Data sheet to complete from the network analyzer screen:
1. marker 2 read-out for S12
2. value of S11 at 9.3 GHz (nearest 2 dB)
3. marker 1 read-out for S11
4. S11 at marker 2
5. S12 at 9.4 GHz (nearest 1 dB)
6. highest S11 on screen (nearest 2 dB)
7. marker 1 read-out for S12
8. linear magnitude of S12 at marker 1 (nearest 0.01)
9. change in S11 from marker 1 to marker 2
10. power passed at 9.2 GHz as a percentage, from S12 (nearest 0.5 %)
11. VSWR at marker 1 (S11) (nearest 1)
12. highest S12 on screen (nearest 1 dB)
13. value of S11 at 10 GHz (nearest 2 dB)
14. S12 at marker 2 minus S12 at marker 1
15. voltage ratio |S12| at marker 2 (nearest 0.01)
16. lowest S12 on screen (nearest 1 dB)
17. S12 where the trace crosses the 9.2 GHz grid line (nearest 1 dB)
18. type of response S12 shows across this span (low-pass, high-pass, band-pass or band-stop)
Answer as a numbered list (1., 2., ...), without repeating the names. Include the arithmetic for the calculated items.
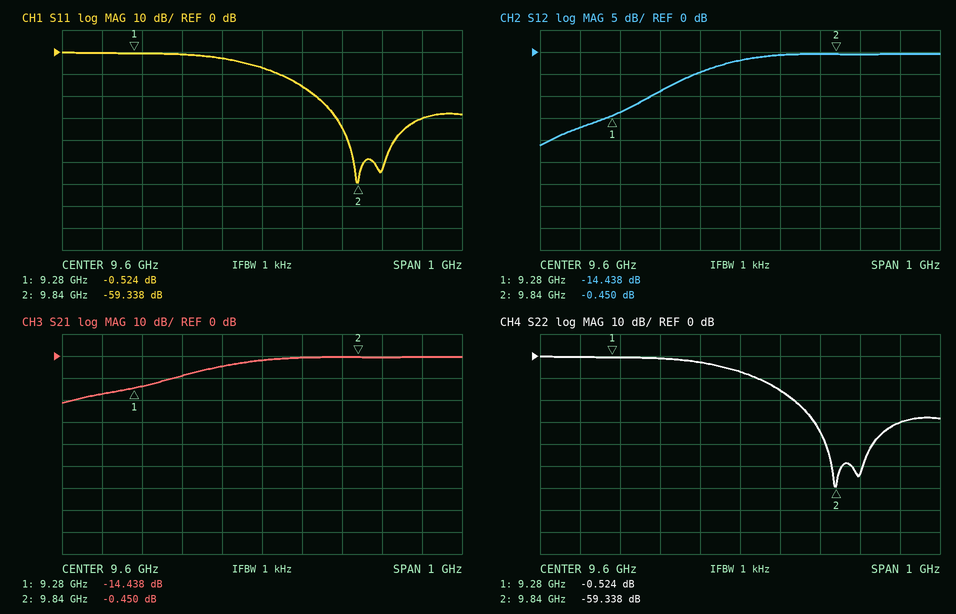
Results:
1. -0.450 dB
2. 0 dB
3. -0.524 dB
4. -59.338 dB
5. -9 dB
6. 0 dB
7. -14.438 dB
8. 10^(-14.438/20) ≈ 0.19
9. -59.338 − (-0.524) = -58.814 dB
10. 10^(-17/10) ≈ 2.0 %
11. (1 + 0.9415)/(1 − 0.9415) ≈ 33
12. 0 dB
13. -30 dB
14. -0.45 − (-14.438) = 13.988 dB
15. 10^(-0.45/20) ≈ 0.95
16. -21 dB
17. -17 dB
18. high-pass
